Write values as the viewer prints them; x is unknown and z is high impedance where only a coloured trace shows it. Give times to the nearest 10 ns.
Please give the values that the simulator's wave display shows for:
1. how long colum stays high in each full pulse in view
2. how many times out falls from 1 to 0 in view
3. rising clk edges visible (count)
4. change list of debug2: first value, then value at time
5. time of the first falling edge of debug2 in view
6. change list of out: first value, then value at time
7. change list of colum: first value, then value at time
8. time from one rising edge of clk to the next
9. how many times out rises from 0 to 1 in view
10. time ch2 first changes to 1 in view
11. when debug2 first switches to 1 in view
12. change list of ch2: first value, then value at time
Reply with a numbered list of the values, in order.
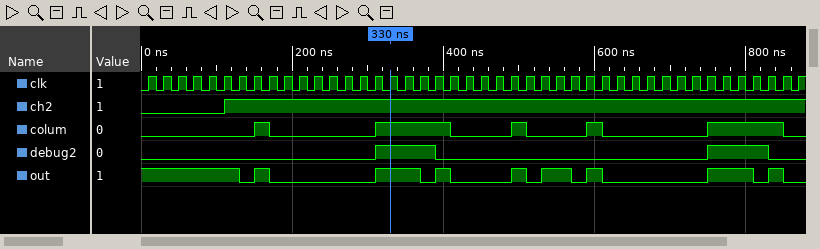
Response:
1. 20 ns, 100 ns, 20 ns, 20 ns, 100 ns
2. 9
3. 44
4. 0, 1 at 310 ns, 0 at 390 ns, 1 at 750 ns, 0 at 830 ns
5. 390 ns
6. 1, 0 at 130 ns, 1 at 150 ns, 0 at 170 ns, 1 at 310 ns, 0 at 370 ns, 1 at 390 ns, 0 at 410 ns, 1 at 490 ns, 0 at 510 ns, 1 at 530 ns, 0 at 570 ns, 1 at 590 ns, 0 at 610 ns, 1 at 750 ns, 0 at 810 ns, 1 at 830 ns, 0 at 850 ns
7. 0, 1 at 150 ns, 0 at 170 ns, 1 at 310 ns, 0 at 410 ns, 1 at 490 ns, 0 at 510 ns, 1 at 590 ns, 0 at 610 ns, 1 at 750 ns, 0 at 850 ns
8. 20 ns
9. 8
10. 110 ns
11. 310 ns
12. 0, 1 at 110 ns
